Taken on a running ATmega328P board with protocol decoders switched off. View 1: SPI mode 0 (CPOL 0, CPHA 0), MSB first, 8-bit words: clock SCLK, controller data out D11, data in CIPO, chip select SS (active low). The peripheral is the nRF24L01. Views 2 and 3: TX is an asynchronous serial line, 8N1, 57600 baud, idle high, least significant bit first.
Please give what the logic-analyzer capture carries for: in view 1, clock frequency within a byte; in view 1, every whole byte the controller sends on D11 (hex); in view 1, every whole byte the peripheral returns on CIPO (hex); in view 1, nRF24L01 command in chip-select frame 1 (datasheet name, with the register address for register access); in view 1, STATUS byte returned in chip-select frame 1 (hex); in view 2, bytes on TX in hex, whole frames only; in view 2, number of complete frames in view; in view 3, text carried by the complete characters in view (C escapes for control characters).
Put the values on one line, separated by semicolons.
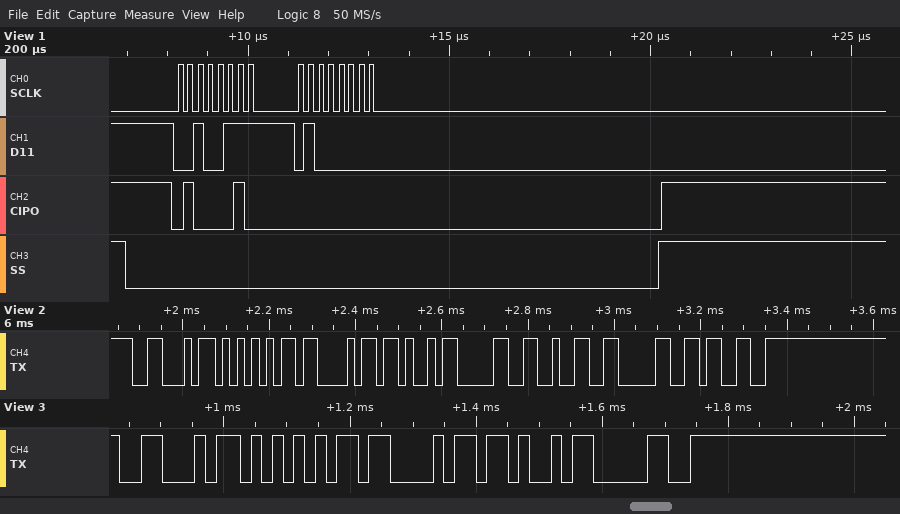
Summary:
4 MHz; 27 40; 42 00; W_REGISTER 0x07; 0x42; 46 55 43 4B 30 32 30 33; 8; "FUCK0"
